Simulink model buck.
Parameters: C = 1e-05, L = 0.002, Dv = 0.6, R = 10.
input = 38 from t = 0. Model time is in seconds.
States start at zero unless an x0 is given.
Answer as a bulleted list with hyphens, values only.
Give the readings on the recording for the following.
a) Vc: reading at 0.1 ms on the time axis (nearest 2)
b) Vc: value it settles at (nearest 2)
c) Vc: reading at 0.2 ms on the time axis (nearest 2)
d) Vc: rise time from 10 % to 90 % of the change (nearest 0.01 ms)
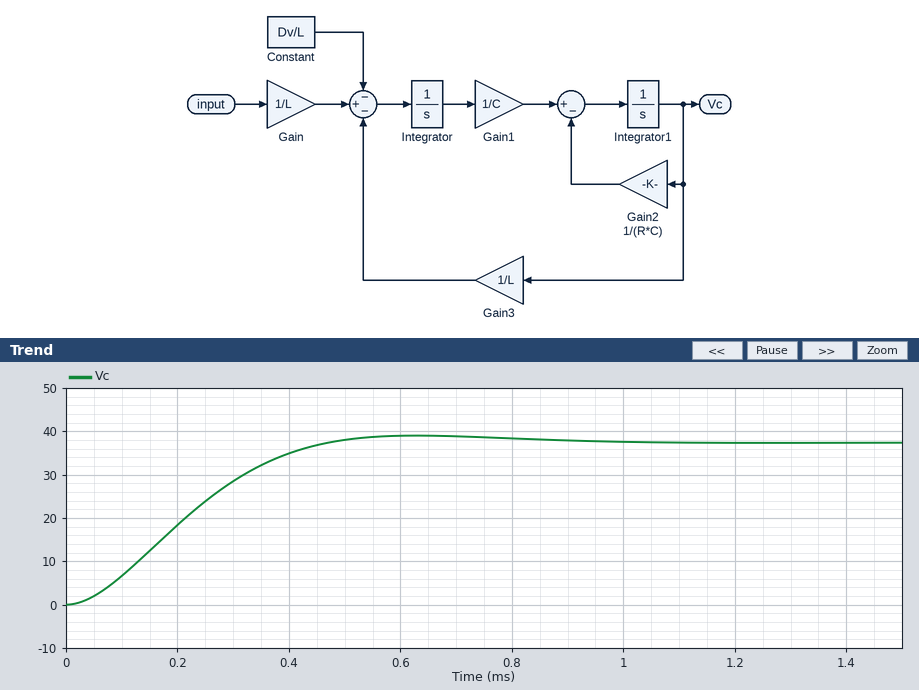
- 6
- 38
- 18
- 0.30 ms
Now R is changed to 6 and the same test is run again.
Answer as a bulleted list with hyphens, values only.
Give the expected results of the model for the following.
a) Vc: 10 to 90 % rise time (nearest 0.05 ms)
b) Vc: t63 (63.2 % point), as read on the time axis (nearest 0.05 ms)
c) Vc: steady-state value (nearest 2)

- 0.60 ms
- 0.35 ms
- 38
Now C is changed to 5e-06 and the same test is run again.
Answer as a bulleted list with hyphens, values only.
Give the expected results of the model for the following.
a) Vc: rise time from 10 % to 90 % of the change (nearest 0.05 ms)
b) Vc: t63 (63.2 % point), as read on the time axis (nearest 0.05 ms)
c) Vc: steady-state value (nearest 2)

- 0.35 ms
- 0.20 ms
- 38
